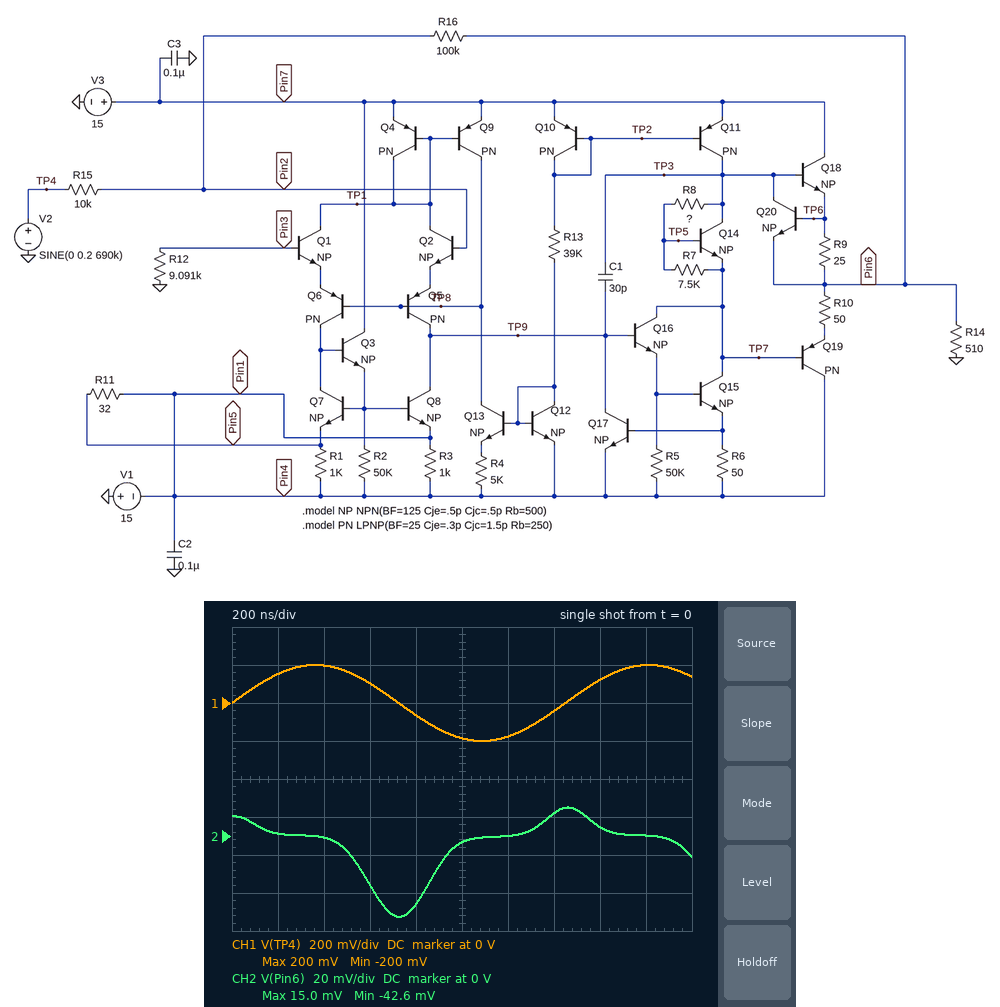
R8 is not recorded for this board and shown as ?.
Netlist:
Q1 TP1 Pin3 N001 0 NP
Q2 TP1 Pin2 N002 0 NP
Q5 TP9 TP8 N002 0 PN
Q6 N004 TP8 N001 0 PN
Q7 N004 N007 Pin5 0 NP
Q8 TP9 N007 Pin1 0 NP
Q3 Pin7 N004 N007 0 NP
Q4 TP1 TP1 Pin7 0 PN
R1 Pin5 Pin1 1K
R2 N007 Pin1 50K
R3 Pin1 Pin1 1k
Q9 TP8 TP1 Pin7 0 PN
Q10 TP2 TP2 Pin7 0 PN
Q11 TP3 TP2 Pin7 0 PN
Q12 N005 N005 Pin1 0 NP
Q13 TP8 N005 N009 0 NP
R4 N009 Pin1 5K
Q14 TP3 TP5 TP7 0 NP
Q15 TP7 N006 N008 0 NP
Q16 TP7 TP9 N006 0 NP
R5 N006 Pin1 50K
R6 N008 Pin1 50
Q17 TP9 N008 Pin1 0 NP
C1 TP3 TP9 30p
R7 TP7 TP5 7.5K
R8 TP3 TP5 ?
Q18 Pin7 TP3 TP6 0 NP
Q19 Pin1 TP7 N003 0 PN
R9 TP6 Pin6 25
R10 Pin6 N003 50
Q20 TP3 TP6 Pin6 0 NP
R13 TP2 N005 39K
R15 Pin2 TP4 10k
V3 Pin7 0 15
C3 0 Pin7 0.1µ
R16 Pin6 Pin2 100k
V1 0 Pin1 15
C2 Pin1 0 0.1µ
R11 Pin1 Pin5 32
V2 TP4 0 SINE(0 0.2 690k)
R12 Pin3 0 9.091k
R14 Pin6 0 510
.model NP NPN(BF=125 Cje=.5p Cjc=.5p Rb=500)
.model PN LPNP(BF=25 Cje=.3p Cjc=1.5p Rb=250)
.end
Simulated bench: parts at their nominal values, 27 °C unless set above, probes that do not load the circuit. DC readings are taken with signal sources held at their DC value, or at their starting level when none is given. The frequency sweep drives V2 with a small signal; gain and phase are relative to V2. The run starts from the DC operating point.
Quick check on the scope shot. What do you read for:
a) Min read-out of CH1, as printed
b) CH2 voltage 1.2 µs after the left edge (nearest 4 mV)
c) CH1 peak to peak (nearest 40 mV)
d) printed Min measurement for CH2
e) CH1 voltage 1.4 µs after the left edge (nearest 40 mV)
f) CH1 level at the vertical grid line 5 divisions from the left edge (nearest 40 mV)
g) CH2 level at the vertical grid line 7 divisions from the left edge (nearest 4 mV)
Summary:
-200 mV
0 V
400 mV
-42.6 mV
-40 mV
-200 mV
12 mV
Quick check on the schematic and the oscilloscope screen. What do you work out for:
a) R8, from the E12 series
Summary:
3.3 kΩ
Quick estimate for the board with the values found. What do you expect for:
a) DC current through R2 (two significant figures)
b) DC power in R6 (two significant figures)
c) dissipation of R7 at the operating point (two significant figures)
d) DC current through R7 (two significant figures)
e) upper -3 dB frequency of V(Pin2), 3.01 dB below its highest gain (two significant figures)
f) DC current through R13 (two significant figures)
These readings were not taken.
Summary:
13 µA
22 µW
77 µW
100 µA
29 MHz
730 µA
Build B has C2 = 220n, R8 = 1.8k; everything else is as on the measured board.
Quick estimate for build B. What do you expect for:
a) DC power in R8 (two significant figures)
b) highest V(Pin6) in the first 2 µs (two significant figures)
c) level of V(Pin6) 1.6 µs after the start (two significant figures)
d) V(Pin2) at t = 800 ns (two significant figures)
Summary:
20 µW
13 mV
4.0 mV
-56 mV
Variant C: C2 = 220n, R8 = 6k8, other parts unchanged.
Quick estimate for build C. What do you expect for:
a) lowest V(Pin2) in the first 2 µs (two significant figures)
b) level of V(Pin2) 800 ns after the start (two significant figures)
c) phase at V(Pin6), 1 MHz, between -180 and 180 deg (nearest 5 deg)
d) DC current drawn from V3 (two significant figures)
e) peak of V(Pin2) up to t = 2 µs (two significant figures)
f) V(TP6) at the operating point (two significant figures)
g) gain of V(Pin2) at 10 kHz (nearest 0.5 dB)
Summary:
-190 mV
-77 mV
90 deg
1.7 mA
170 mV
16 mV
-18.5 dB
